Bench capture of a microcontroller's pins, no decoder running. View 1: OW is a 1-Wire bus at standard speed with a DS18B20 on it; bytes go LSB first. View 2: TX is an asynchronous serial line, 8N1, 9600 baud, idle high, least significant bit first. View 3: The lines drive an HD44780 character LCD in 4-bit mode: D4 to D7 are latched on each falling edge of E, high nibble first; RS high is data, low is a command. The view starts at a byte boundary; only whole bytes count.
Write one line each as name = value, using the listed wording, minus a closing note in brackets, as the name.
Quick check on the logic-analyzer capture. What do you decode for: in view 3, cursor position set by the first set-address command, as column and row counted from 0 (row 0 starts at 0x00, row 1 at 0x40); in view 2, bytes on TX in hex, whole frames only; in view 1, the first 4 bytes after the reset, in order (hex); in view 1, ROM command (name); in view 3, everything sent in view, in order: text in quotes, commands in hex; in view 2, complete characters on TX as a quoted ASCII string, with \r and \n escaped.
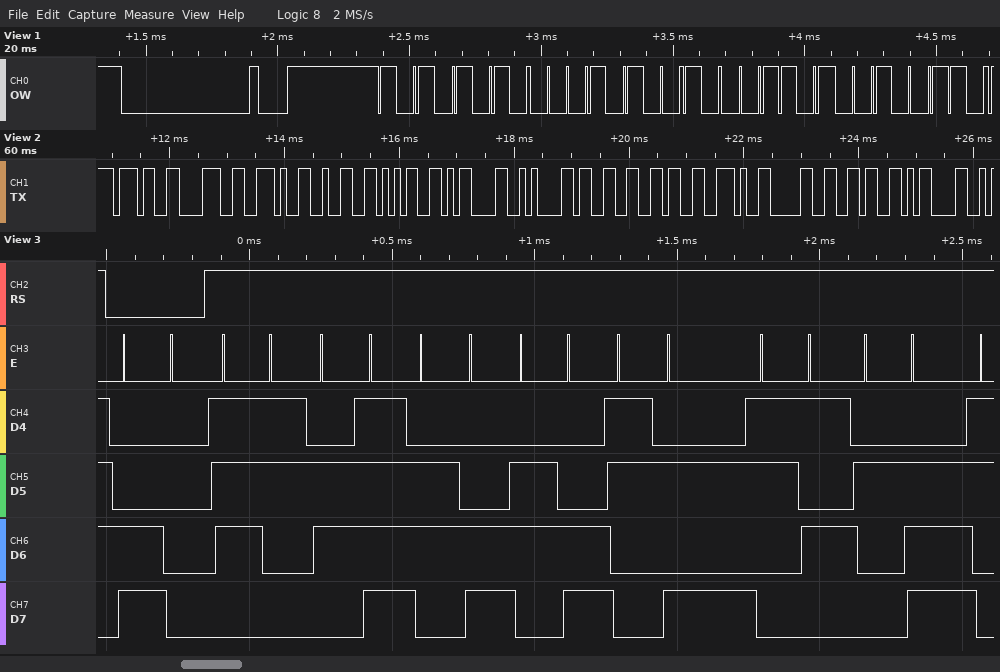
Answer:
in view 3, cursor position set by the first set-address command, as column and row counted from 0 = column 0, row 1
in view 2, bytes on TX in hex, whole frames only = 37 38 2E 32 35 0D 0A 33 36 2E 30 36 0D
in view 1, the first 4 bytes after the reset, in order = 55 28 B1 64
in view 1, ROM command = Match ROM
in view 3, everything sent in view, in order: text in quotes, commands in hex = 0xC0 "soll:5."
in view 2, complete characters on TX as a quoted ASCII string, with \r and \n escaped = "78.25\r\n36.06\r"
